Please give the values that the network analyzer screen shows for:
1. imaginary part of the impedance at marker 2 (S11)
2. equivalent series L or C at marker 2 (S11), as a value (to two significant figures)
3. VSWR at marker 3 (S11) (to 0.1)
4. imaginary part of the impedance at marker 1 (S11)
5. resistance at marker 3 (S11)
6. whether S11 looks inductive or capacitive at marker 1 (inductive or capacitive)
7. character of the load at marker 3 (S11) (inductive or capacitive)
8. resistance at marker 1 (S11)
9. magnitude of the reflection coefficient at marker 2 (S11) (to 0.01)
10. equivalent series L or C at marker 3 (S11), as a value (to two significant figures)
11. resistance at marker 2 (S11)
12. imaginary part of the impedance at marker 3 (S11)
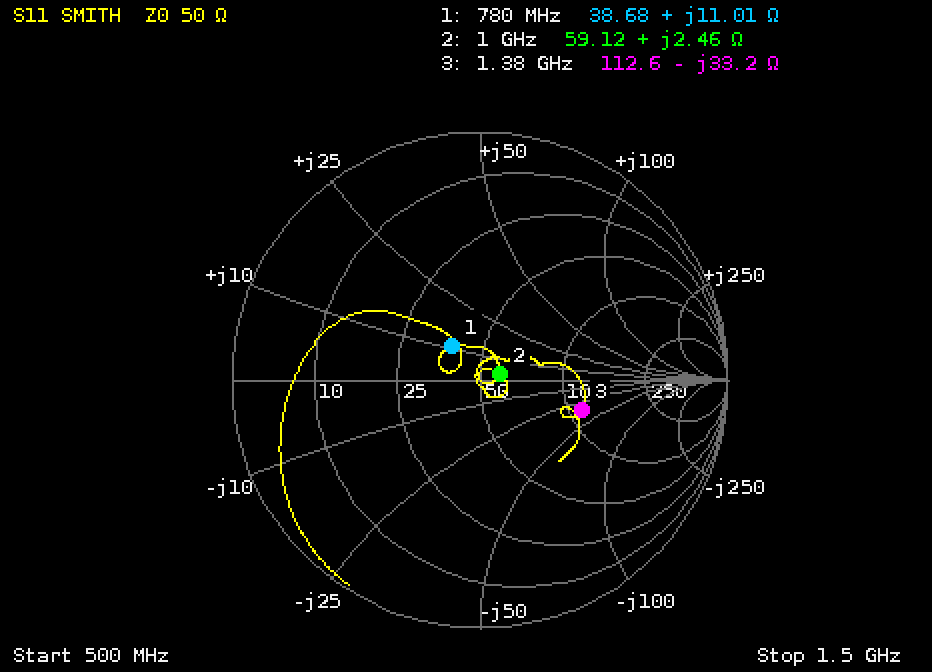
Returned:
+2.46 Ω
390 pH
2.5
+11.01 Ω
112.6 Ω
inductive
capacitive
38.68 Ω
0.09
3.5 pF
59.12 Ω
-33.2 Ω
